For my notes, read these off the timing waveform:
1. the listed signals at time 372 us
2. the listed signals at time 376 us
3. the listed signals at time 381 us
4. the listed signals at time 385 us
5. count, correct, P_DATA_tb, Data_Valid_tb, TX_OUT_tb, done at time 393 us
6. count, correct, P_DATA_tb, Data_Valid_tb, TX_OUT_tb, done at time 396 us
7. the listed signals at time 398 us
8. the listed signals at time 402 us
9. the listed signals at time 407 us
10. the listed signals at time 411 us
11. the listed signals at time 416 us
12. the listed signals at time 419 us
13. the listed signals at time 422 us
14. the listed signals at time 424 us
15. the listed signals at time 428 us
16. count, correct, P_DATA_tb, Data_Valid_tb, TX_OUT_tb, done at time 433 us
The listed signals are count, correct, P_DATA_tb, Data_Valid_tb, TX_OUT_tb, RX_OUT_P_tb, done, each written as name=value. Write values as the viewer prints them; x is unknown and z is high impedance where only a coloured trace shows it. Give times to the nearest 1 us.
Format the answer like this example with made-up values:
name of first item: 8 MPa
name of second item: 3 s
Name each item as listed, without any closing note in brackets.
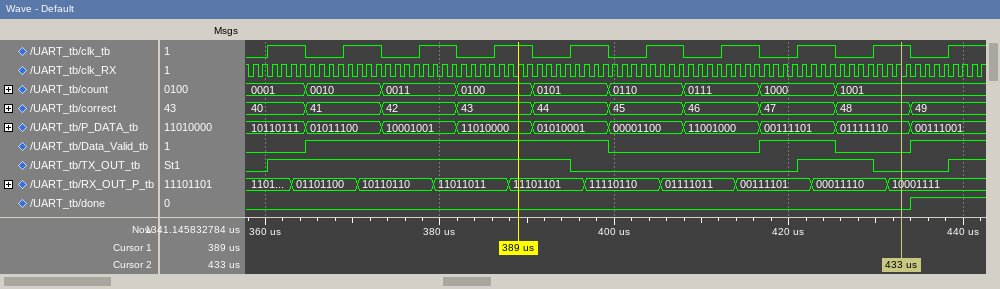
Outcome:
the listed signals at time 372 us: count=0010, correct=41, P_DATA_tb=01011100, Data_Valid_tb=1, TX_OUT_tb=1, RX_OUT_P_tb=10110110, done=0
the listed signals at time 376 us: count=0011, correct=42, P_DATA_tb=10001001, Data_Valid_tb=1, TX_OUT_tb=1, RX_OUT_P_tb=10110110, done=0
the listed signals at time 381 us: count=0011, correct=42, P_DATA_tb=10001001, Data_Valid_tb=1, TX_OUT_tb=1, RX_OUT_P_tb=11011011, done=0
the listed signals at time 385 us: count=0100, correct=43, P_DATA_tb=11010000, Data_Valid_tb=1, TX_OUT_tb=1, RX_OUT_P_tb=11011011, done=0
count, correct, P_DATA_tb, Data_Valid_tb, TX_OUT_tb, done at time 393 us: count=0101, correct=44, P_DATA_tb=01010001, Data_Valid_tb=1, TX_OUT_tb=1, done=0
count, correct, P_DATA_tb, Data_Valid_tb, TX_OUT_tb, done at time 396 us: count=0101, correct=44, P_DATA_tb=01010001, Data_Valid_tb=1, TX_OUT_tb=0, done=0
the listed signals at time 398 us: count=0101, correct=44, P_DATA_tb=01010001, Data_Valid_tb=1, TX_OUT_tb=0, RX_OUT_P_tb=11110110, done=0
the listed signals at time 402 us: count=0110, correct=45, P_DATA_tb=00001100, Data_Valid_tb=0, TX_OUT_tb=0, RX_OUT_P_tb=11110110, done=0
the listed signals at time 407 us: count=0110, correct=45, P_DATA_tb=00001100, Data_Valid_tb=0, TX_OUT_tb=0, RX_OUT_P_tb=01111011, done=0
the listed signals at time 411 us: count=0111, correct=46, P_DATA_tb=11001000, Data_Valid_tb=0, TX_OUT_tb=0, RX_OUT_P_tb=01111011, done=0
the listed signals at time 416 us: count=0111, correct=46, P_DATA_tb=11001000, Data_Valid_tb=0, TX_OUT_tb=0, RX_OUT_P_tb=00111101, done=0
the listed signals at time 419 us: count=1000, correct=47, P_DATA_tb=00111101, Data_Valid_tb=1, TX_OUT_tb=0, RX_OUT_P_tb=00111101, done=0
the listed signals at time 422 us: count=1000, correct=47, P_DATA_tb=00111101, Data_Valid_tb=1, TX_OUT_tb=1, RX_OUT_P_tb=00111101, done=0
the listed signals at time 424 us: count=1000, correct=47, P_DATA_tb=00111101, Data_Valid_tb=1, TX_OUT_tb=1, RX_OUT_P_tb=00011110, done=0
the listed signals at time 428 us: count=1001, correct=48, P_DATA_tb=01111110, Data_Valid_tb=0, TX_OUT_tb=1, RX_OUT_P_tb=00011110, done=0
count, correct, P_DATA_tb, Data_Valid_tb, TX_OUT_tb, done at time 433 us: count=1001, correct=48, P_DATA_tb=01111110, Data_Valid_tb=0, TX_OUT_tb=0, done=0
